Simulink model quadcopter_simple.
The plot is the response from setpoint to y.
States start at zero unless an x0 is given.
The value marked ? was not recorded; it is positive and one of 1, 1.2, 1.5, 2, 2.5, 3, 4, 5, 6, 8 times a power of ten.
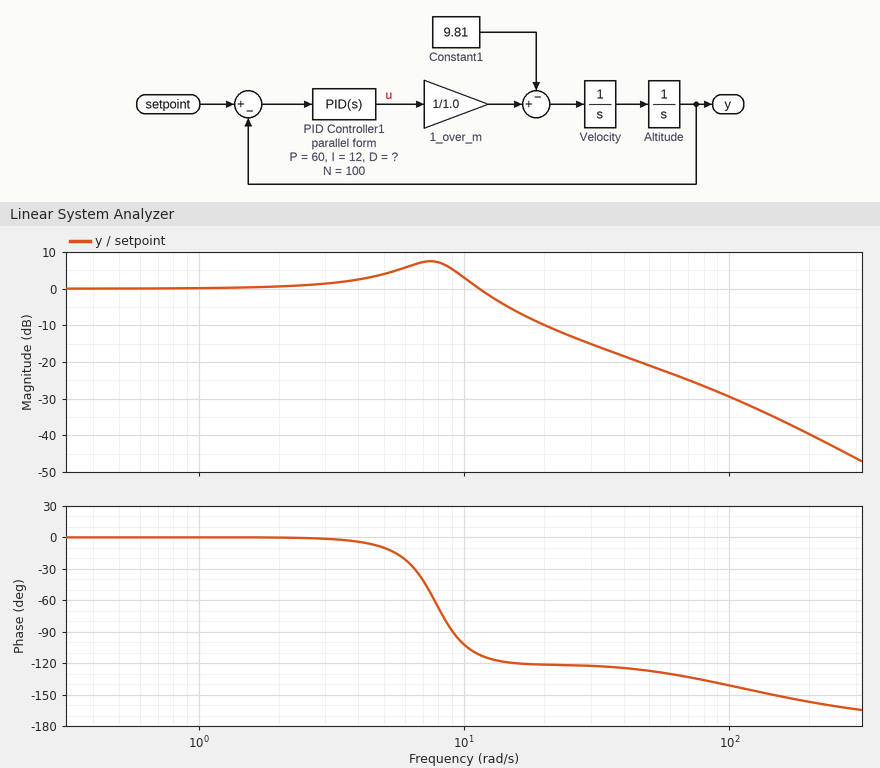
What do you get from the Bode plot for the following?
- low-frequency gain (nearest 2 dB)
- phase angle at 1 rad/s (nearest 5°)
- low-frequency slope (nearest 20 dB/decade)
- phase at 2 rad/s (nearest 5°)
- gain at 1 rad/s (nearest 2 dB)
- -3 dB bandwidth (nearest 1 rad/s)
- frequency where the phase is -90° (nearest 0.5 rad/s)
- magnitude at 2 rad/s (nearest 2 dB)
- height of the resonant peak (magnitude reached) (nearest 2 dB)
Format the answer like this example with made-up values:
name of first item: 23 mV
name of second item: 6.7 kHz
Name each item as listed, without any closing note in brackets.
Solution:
low-frequency gain: 0 dB
phase angle at 1 rad/s: 0°
low-frequency slope: 0 dB/decade
phase at 2 rad/s: 0°
gain at 1 rad/s: 0 dB
-3 dB bandwidth: 13 rad/s
frequency where the phase is -90°: 9.0 rad/s
magnitude at 2 rad/s: 0 dB
height of the resonant peak (magnitude reached): 8 dB
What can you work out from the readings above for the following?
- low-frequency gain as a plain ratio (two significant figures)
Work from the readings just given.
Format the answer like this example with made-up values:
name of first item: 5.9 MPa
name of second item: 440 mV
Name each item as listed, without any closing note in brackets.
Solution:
low-frequency gain as a plain ratio: 1.0
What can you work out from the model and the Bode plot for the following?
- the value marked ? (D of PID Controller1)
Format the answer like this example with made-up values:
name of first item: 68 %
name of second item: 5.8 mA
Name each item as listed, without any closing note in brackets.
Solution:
the value marked ?: 4
